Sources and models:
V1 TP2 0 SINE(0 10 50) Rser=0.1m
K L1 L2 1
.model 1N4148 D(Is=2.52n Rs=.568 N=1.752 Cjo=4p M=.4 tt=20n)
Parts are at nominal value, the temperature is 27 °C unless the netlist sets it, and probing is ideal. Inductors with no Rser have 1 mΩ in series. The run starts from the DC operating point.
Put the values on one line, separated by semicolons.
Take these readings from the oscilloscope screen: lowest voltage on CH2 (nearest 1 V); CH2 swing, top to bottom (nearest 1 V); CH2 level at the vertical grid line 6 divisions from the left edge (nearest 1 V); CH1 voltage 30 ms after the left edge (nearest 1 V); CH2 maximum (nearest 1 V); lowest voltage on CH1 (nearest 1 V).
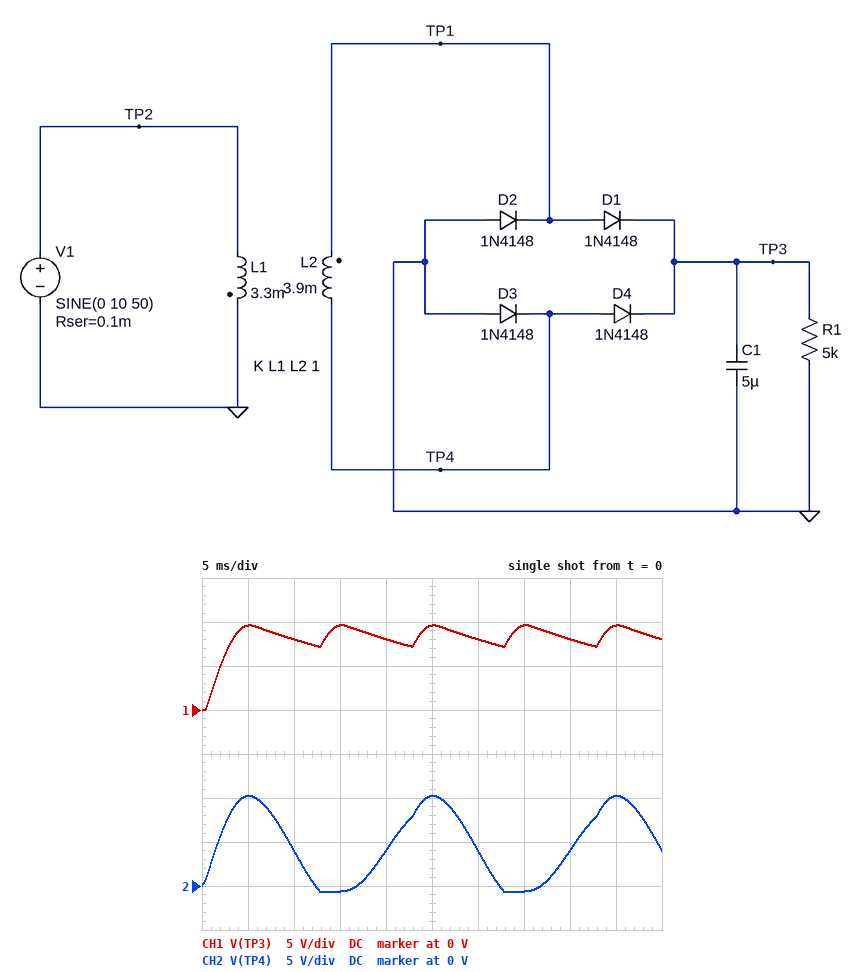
-1 V; 11 V; 4 V; 8 V; 10 V; 0 V
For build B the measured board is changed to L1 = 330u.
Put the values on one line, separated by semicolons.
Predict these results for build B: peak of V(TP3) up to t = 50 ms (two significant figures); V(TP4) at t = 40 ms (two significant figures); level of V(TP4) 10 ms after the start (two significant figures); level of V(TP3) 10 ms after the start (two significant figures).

33 V; 14 V; 13 V; 27 V
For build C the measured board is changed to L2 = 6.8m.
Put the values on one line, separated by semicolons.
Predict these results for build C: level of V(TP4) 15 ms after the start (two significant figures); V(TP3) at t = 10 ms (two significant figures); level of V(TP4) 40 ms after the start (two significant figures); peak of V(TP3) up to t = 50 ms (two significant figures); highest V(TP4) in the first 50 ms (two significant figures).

-640 mV; 11 V; 5.5 V; 13 V; 14 V
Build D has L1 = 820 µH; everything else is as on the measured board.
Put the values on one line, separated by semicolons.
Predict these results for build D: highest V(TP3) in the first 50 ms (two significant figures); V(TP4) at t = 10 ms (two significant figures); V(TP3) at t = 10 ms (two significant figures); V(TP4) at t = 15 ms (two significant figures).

21 V; 8.4 V; 17 V; -660 mV
